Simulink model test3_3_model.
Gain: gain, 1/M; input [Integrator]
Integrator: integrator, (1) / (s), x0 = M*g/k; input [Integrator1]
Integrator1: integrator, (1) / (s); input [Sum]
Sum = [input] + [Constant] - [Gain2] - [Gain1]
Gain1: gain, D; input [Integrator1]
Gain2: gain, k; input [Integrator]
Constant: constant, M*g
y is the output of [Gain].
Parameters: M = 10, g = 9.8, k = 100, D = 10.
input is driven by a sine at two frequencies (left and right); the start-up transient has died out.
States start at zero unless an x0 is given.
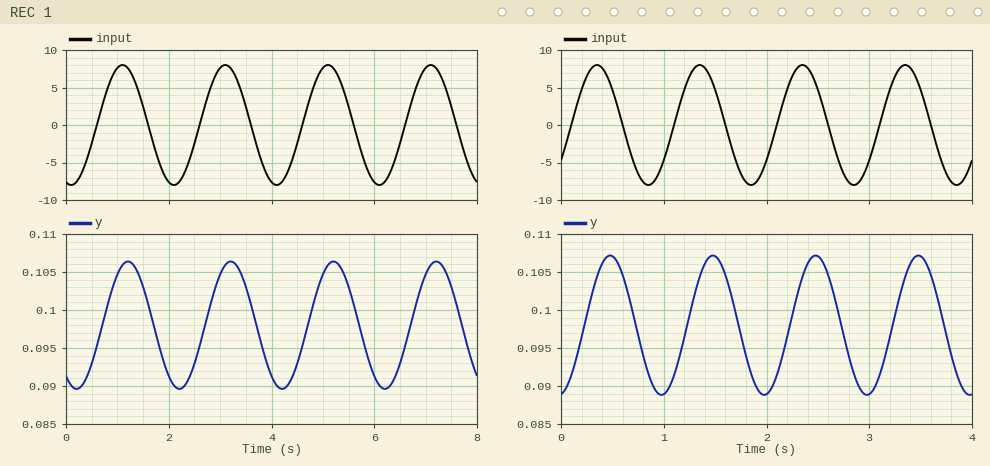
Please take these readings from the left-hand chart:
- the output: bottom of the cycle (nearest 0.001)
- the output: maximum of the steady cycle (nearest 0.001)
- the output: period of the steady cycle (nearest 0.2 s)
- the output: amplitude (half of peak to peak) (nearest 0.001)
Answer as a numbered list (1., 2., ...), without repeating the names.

1. 0.090
2. 0.106
3. 2.0 s
4. 0.008
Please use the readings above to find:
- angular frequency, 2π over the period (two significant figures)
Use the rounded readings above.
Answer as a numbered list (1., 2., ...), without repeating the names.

1. 3.1 rad/s
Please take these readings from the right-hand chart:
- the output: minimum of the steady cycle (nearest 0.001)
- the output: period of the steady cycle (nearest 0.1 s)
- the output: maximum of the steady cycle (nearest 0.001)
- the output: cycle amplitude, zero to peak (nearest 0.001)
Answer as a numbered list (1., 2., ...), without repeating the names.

1. 0.089
2. 1.0 s
3. 0.107
4. 0.009
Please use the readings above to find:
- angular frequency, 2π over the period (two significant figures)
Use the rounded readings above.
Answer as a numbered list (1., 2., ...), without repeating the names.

1. 6.3 rad/s
